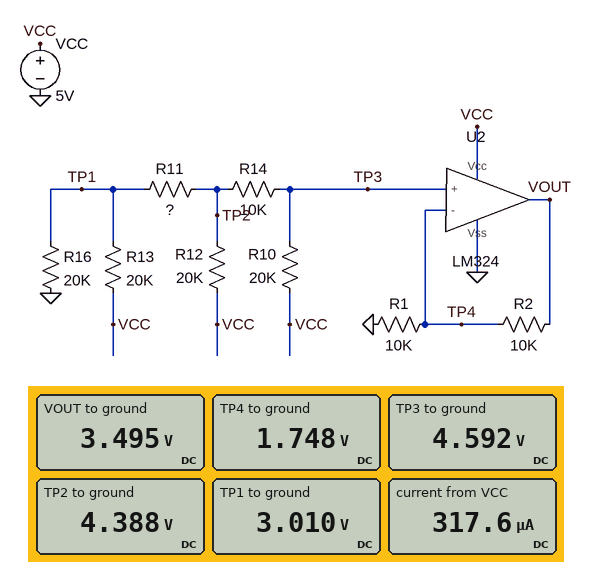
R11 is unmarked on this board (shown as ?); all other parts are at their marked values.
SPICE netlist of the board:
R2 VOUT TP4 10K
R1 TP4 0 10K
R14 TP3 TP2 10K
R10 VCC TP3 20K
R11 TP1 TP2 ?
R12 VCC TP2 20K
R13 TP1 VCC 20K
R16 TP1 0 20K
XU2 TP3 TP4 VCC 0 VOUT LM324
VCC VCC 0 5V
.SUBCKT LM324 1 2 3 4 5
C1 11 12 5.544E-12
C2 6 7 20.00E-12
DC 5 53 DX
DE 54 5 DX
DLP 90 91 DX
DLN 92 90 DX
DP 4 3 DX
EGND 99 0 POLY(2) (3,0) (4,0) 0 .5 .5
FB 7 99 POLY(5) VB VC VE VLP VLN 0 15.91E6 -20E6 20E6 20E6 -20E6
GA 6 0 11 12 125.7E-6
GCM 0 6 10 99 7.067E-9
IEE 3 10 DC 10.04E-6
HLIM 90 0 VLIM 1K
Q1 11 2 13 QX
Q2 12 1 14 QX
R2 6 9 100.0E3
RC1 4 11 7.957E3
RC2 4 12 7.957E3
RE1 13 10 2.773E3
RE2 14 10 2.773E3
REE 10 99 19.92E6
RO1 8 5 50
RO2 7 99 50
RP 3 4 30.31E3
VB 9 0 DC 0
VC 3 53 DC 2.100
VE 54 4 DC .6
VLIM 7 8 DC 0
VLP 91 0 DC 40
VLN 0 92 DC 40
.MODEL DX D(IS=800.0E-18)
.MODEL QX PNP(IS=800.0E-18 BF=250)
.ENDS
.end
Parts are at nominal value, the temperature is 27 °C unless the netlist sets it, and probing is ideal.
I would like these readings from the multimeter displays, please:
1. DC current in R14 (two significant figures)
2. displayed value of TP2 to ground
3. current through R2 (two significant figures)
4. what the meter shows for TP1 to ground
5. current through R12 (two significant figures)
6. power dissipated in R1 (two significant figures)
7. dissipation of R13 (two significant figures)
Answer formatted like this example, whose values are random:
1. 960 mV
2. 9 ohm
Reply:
1. 20 µA
2. 4.388 V
3. 170 µA
4. 3.010 V
5. 31 µA
6. 310 µW
7. 200 µW
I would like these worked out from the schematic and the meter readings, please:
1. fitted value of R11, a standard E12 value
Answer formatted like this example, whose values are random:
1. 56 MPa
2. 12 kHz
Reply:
1. 27 kΩ
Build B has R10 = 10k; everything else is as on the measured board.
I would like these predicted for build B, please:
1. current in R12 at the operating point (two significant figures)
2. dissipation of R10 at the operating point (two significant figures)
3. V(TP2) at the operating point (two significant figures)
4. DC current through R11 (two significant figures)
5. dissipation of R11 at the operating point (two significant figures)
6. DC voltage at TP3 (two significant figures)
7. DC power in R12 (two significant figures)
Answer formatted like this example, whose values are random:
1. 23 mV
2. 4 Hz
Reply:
1. 27 µA
2. 7.1 µW
3. 4.5 V
4. 53 µA
5. 76 µW
6. 4.7 V
7. 14 µW
